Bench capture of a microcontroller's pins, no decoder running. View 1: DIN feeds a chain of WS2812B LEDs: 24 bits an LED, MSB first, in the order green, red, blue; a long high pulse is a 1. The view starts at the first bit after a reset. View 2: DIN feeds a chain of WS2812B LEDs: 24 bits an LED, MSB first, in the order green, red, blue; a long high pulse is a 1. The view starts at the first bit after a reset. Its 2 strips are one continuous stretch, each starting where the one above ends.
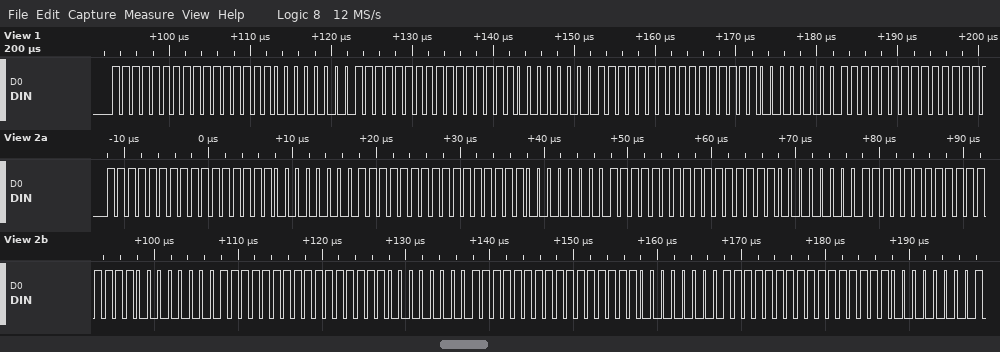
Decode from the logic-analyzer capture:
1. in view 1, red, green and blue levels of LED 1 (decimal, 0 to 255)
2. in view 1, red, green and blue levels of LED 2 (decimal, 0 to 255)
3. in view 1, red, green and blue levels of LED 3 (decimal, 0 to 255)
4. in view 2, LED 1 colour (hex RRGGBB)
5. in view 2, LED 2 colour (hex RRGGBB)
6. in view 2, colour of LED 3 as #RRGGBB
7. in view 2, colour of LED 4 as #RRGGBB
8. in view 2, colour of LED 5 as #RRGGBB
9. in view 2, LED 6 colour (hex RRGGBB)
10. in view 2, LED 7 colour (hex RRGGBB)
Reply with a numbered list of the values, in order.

1. 255, 255, 0
2. 255, 255, 0
3. 255, 255, 0
4. #FFFF00
5. #FFFF00
6. #FFFF00
7. #FFFF00
8. #FFFF00
9. #FFFF00
10. #FFFF00
